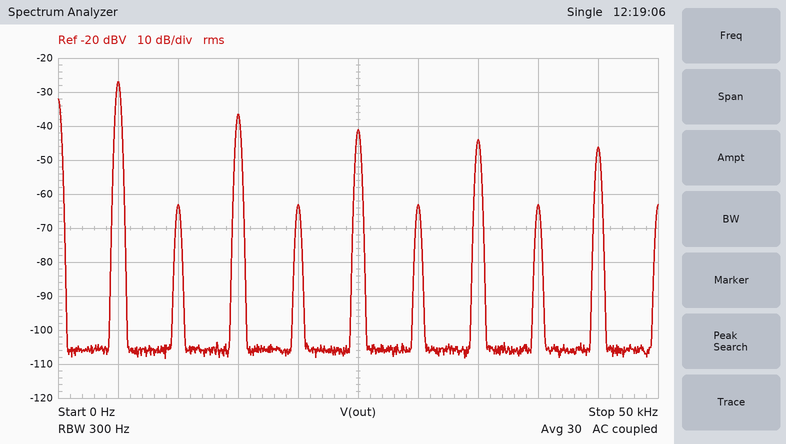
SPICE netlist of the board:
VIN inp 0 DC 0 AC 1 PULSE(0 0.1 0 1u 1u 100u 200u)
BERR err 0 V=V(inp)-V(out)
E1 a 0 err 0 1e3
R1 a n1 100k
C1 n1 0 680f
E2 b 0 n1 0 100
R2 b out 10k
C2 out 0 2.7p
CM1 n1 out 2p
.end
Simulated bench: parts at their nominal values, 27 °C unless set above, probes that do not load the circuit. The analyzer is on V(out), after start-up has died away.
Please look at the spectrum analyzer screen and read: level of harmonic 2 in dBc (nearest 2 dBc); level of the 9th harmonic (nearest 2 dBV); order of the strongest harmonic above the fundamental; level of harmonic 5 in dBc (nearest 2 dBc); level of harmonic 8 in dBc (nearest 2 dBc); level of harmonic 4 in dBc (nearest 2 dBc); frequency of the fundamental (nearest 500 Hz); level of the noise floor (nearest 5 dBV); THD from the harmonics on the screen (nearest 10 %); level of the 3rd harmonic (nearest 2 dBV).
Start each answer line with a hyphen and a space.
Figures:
- -36 dBc
- -46 dBV
- 3
- -14 dBc
- -36 dBc
- -36 dBc
- 5.0 kHz
- -105 dBV
- 40 %
- -36 dBV
